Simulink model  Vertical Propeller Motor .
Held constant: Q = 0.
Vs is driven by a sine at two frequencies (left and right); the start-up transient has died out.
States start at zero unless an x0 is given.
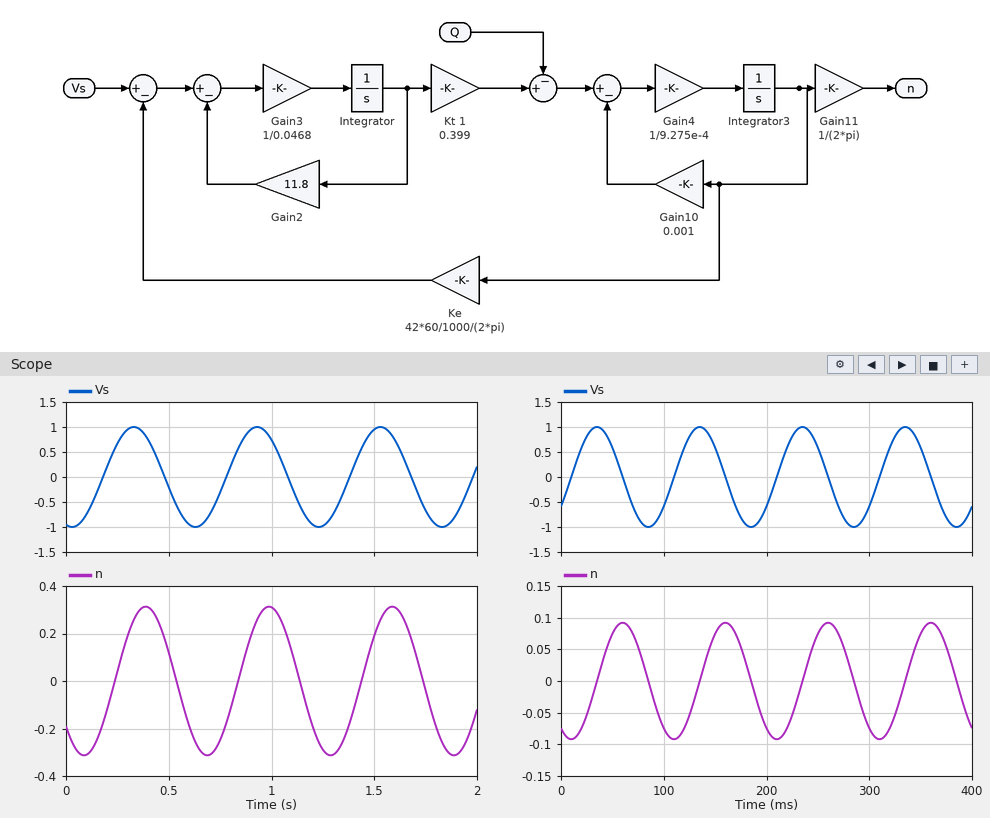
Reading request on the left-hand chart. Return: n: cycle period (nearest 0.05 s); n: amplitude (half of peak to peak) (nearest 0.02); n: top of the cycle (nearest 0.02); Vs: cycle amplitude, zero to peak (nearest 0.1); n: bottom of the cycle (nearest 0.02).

0.60 s
0.32
0.32
1.0
-0.32
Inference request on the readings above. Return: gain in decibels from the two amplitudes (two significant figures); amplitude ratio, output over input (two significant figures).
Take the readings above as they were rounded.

-9.9 dB
0.32
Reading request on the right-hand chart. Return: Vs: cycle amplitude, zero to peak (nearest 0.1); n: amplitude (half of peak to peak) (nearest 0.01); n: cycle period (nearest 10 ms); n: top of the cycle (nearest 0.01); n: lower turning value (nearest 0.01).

1.0
0.09
100 ms
0.09
-0.09
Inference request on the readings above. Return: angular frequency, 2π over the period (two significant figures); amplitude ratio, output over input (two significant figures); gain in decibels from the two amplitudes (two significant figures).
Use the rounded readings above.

0.063 rad/ms
0.090
-21 dB
